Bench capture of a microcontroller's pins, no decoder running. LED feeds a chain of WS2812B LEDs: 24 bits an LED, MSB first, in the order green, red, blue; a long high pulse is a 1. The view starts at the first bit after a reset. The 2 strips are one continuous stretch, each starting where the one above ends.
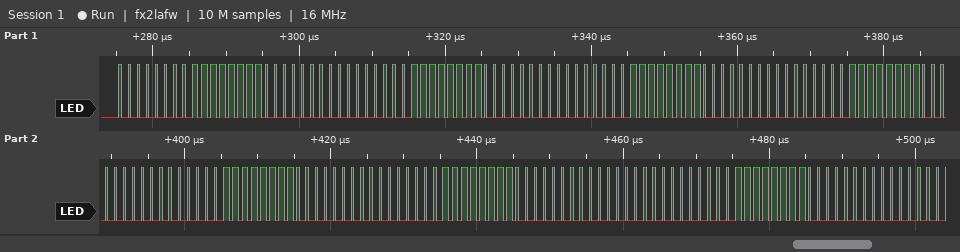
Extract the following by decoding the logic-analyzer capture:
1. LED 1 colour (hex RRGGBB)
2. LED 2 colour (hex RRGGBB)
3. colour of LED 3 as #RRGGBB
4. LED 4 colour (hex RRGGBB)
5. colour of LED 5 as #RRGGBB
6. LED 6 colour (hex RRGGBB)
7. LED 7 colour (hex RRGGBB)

#FF0000
#FF0000
#FF0000
#FF0000
#FF0000
#FF0000
#0000FF
